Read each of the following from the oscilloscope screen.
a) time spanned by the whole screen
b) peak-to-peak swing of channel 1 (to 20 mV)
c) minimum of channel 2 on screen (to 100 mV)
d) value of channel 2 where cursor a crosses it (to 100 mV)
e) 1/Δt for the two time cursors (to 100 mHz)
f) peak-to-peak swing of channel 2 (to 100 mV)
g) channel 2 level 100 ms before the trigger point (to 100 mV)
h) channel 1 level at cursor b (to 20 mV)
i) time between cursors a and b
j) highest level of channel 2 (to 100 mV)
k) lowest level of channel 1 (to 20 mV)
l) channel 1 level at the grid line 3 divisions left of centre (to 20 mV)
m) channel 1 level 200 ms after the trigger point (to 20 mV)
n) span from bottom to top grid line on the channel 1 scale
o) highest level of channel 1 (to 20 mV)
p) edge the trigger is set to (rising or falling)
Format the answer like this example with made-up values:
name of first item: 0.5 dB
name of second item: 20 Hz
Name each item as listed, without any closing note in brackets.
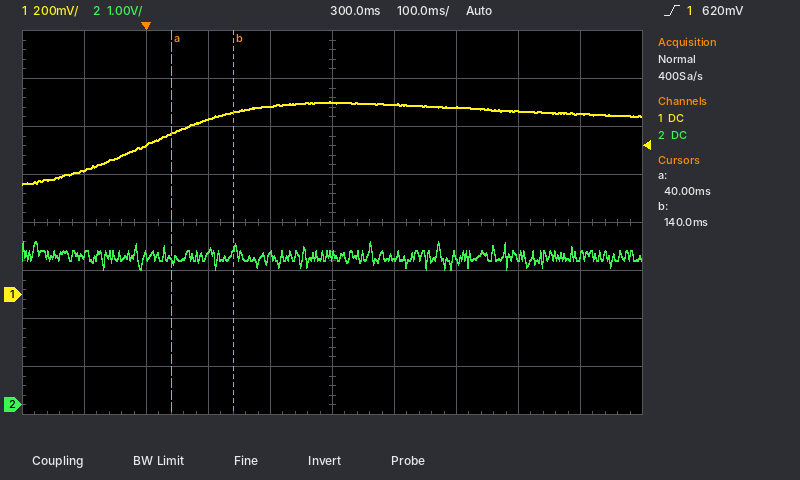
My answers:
time spanned by the whole screen: 1 s
peak-to-peak swing of channel 1: 340 mV
minimum of channel 2 on screen: 2.8 V
value of channel 2 where cursor a crosses it: 3.0 V
1/Δt for the two time cursors: 10.0 Hz
peak-to-peak swing of channel 2: 600 mV
channel 2 level 100 ms before the trigger point: 3.1 V
channel 1 level at cursor b: 760 mV
time between cursors a and b: 100 ms
highest level of channel 2: 3.4 V
lowest level of channel 1: 460 mV
channel 1 level at the grid line 3 divisions left of centre: 620 mV
channel 1 level 200 ms after the trigger point: 780 mV
span from bottom to top grid line on the channel 1 scale: 1.6 V
highest level of channel 1: 800 mV
edge the trigger is set to: rising
